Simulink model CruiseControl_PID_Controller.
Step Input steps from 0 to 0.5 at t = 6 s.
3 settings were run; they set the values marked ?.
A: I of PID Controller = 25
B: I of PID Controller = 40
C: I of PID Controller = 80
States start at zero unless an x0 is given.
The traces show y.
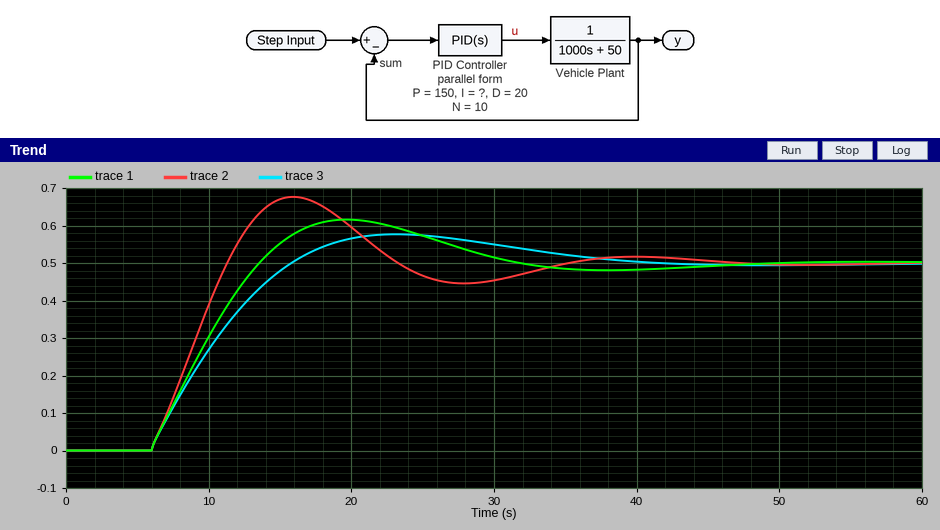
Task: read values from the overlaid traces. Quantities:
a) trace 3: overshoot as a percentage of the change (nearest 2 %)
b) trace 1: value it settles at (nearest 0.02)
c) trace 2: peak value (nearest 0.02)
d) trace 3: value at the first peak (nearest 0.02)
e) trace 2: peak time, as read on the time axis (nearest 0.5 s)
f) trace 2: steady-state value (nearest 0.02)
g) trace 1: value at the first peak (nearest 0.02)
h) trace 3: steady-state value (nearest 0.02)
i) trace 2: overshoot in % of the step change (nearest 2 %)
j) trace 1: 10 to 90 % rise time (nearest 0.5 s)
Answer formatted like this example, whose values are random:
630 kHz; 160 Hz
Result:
16 %; 0.50; 0.68; 0.58; 16.0 s; 0.50; 0.62; 0.50; 36 %; 6.0 s
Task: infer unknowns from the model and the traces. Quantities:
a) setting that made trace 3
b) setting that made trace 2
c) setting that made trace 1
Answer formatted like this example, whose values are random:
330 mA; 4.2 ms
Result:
A; C; B
